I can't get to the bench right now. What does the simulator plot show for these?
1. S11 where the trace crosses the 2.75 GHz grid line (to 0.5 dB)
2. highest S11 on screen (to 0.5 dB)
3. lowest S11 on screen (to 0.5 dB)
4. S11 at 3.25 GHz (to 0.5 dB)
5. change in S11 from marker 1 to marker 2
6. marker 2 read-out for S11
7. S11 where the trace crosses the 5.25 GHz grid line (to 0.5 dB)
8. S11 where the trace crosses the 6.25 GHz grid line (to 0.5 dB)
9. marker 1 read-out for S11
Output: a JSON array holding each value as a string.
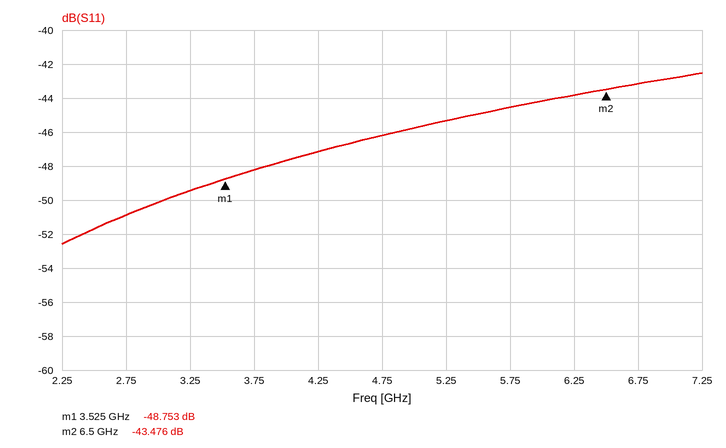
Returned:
["-51.0 dB", "-42.5 dB", "-52.5 dB", "-49.5 dB", "5.277 dB", "-43.476 dB", "-45.5 dB", "-44.0 dB", "-48.753 dB"]
